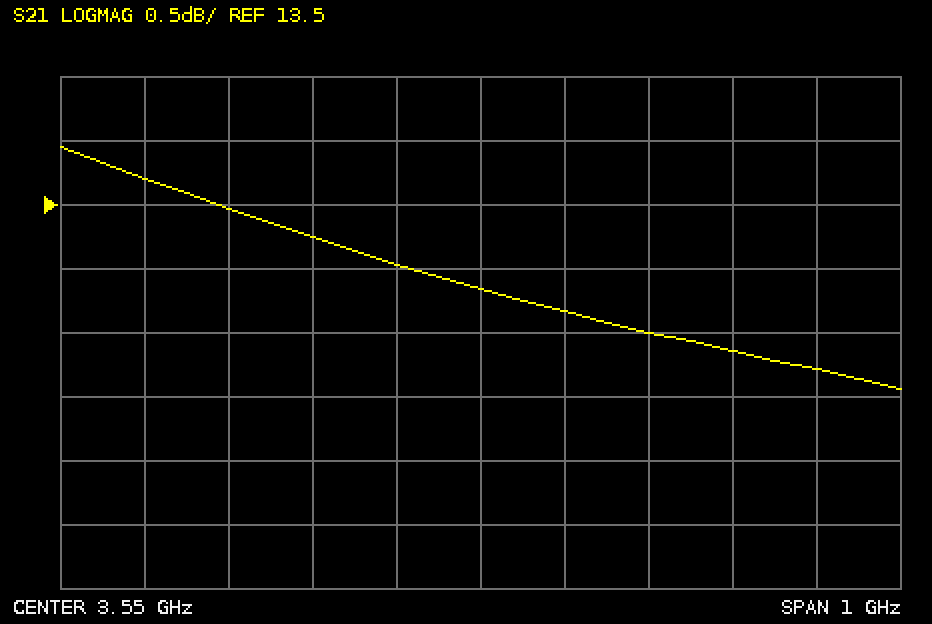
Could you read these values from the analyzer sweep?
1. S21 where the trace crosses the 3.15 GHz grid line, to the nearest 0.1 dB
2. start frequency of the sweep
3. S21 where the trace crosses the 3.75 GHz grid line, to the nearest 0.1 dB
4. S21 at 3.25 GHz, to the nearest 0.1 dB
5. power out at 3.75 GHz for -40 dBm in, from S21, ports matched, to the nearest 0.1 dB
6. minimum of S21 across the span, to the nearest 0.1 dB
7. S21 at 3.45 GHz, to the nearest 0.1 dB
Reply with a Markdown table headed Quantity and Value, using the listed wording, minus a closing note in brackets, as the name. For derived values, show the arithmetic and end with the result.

| Quantity | Value |
|---|---|
| S21 where the trace crosses the 3.15 GHz grid line, to the nearest 0.1 dB | 13.7 dB |
| start frequency of the sweep | 3.05 GHz |
| S21 where the trace crosses the 3.75 GHz grid line, to the nearest 0.1 dB | 12.5 dB |
| S21 at 3.25 GHz, to the nearest 0.1 dB | 13.5 dB |
| power out at 3.75 GHz for -40 dBm in, from S21, ports matched, to the nearest 0.1 dB | -40 dBm + (12.5 dB) = -27.5 dBm |
| minimum of S21 across the span, to the nearest 0.1 dB | 12.1 dB |
| S21 at 3.45 GHz, to the nearest 0.1 dB | 13.0 dB |
